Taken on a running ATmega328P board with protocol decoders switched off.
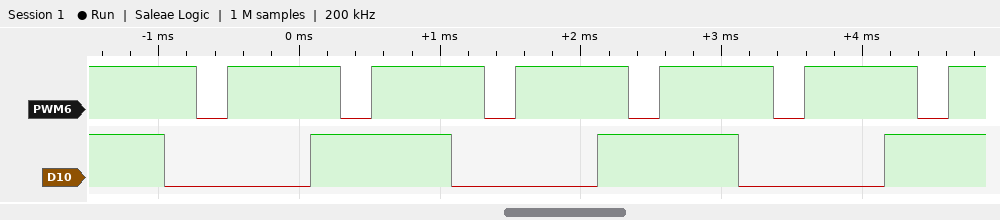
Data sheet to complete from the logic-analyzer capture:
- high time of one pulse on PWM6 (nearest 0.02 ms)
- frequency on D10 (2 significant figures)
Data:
0.80 ms
490 Hz
